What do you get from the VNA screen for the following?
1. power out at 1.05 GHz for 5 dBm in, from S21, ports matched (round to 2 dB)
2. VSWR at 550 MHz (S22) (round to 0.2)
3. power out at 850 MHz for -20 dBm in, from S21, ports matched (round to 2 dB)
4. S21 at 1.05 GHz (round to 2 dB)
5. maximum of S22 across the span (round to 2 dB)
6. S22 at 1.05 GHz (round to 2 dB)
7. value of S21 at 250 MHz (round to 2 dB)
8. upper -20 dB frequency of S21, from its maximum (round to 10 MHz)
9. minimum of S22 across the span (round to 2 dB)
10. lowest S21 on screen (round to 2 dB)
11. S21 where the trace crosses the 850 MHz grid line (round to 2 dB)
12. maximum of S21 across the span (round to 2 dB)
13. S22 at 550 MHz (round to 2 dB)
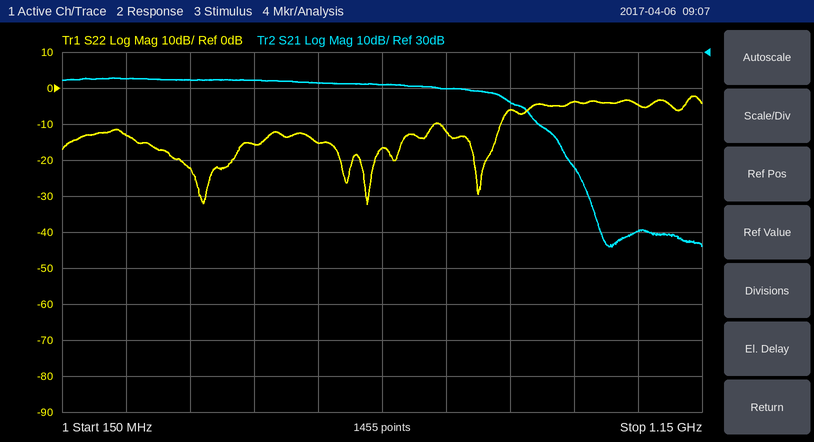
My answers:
-14 dBm
1.4
-4 dBm
-20 dB
-2 dB
-4 dB
22 dB
930 MHz
-32 dB
-24 dB
16 dB
22 dB
-16 dB
